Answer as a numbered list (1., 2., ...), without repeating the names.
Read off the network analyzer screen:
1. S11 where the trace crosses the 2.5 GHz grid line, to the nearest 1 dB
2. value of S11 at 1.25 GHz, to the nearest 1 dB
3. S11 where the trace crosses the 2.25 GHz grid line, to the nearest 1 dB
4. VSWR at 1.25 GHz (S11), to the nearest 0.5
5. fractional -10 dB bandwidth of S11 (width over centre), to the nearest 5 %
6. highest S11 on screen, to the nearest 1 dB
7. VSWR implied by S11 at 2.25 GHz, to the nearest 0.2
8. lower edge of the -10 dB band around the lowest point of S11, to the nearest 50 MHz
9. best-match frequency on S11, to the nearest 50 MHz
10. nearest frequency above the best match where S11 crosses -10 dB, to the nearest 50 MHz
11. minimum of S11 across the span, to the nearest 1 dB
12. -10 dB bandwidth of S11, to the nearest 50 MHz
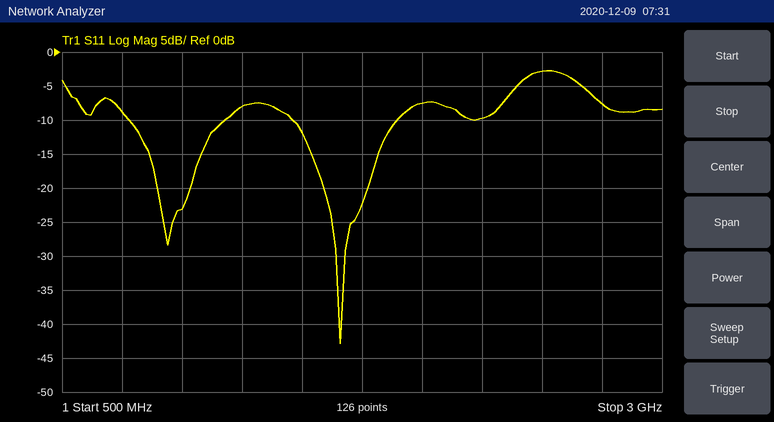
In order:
1. -3 dB
2. -8 dB
3. -10 dB
4. 2.5
5. 25 %
6. -3 dB
7. 2.0
8. 1.45 GHz
9. 1.65 GHz
10. 1.90 GHz
11. -43 dB
12. 450 MHz
